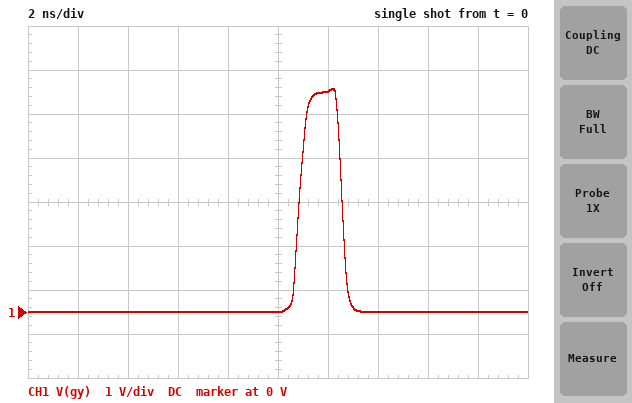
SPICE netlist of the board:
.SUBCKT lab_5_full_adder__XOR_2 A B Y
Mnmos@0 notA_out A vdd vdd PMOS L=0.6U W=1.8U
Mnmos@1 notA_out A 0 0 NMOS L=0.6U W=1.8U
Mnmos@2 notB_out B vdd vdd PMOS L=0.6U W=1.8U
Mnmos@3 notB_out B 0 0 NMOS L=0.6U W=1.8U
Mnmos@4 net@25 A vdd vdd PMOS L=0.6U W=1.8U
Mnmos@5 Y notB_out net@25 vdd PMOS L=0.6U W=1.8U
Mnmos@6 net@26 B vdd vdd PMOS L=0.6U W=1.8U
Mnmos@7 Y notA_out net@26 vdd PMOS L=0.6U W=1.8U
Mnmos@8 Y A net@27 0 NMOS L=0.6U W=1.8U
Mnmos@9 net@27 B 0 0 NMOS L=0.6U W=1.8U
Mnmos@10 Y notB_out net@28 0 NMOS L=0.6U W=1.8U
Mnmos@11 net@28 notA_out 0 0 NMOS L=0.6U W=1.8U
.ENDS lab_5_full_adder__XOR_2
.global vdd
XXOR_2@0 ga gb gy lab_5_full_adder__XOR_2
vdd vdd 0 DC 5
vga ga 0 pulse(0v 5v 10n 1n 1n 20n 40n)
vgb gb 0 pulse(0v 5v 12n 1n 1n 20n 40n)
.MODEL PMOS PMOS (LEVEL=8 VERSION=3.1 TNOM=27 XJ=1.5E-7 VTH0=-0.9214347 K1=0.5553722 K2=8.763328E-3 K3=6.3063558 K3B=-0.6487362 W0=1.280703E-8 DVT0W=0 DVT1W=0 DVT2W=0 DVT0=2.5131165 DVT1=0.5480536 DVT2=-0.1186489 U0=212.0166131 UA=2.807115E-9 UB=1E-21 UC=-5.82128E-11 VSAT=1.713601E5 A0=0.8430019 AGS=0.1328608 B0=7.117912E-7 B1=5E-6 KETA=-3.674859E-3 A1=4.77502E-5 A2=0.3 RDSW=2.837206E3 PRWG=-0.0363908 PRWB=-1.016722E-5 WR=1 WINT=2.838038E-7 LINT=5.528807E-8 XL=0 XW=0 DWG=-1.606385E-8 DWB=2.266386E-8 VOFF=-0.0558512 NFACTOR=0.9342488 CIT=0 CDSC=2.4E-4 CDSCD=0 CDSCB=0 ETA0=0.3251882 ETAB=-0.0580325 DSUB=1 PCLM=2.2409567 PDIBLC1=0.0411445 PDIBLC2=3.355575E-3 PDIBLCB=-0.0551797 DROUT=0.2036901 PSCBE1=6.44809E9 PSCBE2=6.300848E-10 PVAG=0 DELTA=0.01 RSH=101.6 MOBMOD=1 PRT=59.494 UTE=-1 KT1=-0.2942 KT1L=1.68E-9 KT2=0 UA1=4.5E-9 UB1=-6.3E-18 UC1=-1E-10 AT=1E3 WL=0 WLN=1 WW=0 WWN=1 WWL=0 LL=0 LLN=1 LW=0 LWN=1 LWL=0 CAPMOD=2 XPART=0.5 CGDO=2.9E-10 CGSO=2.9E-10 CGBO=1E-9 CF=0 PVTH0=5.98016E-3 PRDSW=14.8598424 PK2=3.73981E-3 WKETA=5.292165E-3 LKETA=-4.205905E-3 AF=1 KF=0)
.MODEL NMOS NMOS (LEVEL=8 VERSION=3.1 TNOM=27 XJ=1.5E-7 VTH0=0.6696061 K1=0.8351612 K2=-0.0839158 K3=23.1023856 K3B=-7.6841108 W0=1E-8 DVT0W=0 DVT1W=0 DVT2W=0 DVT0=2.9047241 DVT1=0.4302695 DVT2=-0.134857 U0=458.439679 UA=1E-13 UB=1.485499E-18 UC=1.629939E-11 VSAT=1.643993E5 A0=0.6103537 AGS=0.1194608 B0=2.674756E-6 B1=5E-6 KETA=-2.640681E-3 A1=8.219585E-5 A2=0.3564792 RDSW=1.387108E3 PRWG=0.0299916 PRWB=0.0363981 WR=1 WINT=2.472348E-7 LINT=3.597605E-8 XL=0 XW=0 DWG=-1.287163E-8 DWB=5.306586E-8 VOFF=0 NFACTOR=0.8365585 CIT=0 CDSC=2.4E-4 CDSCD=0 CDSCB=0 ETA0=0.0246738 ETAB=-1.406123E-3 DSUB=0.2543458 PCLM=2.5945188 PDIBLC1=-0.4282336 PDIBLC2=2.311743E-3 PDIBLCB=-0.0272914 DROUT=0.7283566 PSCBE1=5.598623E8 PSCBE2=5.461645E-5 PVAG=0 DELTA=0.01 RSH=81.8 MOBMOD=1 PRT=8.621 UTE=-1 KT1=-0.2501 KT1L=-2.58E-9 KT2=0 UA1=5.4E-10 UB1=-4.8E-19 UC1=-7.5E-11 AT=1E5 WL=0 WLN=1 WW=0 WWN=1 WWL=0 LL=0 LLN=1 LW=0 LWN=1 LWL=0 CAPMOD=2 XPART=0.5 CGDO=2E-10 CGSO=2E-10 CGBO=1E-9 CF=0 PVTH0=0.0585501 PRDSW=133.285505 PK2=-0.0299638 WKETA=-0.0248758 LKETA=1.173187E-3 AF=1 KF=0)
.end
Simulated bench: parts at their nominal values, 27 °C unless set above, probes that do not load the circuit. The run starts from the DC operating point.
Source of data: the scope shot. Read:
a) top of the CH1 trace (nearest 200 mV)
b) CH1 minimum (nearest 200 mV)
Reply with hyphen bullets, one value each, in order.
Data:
- 5.0 V
- 0 V
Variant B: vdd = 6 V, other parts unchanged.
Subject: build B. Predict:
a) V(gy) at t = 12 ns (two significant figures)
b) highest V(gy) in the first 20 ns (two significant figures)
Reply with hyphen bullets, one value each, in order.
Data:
- 6.0 V
- 6.1 V
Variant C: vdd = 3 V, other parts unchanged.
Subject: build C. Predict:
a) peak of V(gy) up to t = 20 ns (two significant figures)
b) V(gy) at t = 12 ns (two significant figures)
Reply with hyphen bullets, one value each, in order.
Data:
- 3.1 V
- 3.0 V
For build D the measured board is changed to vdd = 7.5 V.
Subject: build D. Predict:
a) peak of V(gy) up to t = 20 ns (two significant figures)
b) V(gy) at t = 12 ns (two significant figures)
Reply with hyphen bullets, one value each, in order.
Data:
- 7.6 V
- 7.5 V
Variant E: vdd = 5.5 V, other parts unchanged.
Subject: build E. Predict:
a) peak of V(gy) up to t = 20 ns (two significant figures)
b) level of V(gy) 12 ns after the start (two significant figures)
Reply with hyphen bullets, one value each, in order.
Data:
- 5.6 V
- 5.5 V
